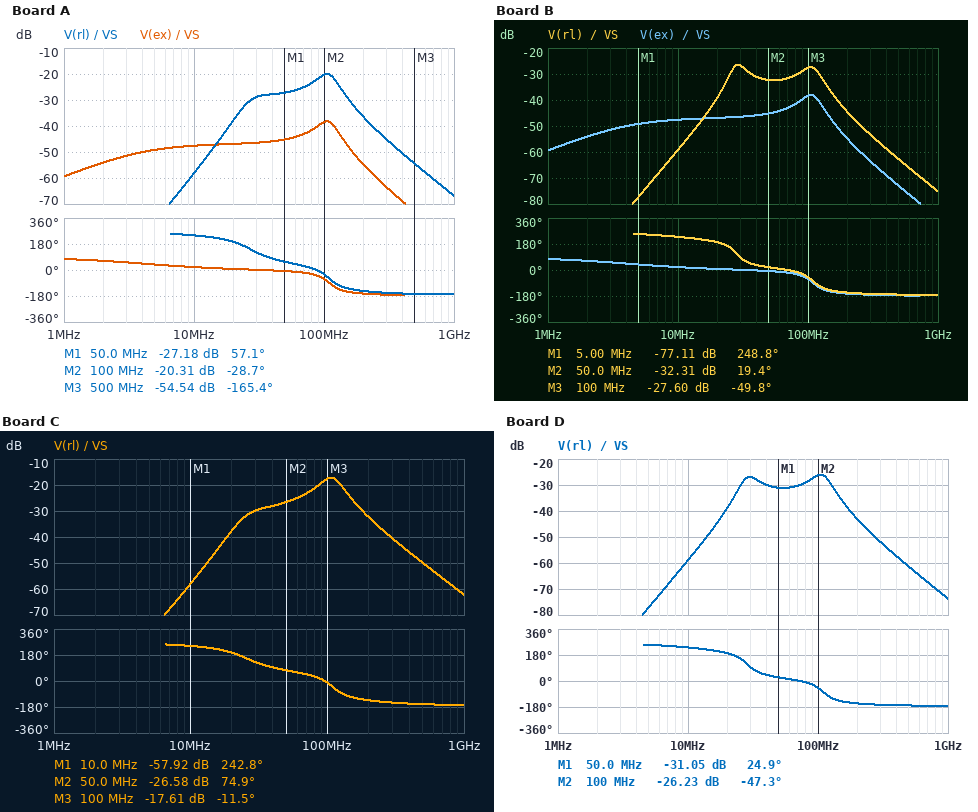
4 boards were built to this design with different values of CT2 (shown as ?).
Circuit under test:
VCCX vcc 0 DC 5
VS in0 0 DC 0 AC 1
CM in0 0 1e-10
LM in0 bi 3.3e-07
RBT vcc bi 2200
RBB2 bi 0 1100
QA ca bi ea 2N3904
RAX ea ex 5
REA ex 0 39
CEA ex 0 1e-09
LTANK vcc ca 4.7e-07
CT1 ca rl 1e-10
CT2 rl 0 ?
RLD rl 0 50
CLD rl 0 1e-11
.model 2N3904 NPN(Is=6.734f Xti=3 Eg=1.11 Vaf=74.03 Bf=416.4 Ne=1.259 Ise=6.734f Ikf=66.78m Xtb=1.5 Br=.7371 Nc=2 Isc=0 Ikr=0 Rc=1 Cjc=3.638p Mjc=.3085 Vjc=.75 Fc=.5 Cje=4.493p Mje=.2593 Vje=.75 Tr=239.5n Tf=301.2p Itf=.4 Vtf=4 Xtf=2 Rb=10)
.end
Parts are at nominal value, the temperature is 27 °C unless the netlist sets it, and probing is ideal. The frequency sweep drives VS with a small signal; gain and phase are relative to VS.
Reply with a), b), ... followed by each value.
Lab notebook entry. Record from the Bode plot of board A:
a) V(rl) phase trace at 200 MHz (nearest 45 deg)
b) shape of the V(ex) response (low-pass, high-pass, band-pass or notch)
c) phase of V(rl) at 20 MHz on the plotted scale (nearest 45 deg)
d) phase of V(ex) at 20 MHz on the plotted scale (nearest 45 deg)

a) -135 deg
b) band-pass
c) 180 deg
d) 0 deg
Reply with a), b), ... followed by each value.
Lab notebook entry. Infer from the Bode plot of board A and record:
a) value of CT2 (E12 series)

a) 39 pF
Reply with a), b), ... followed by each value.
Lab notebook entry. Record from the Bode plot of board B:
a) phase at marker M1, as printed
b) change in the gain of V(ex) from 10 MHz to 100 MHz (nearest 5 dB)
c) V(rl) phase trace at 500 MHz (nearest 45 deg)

a) 248.8 deg
b) 10 dB
c) -180 deg
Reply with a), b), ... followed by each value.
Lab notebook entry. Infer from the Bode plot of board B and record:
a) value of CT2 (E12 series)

a) 120 pF
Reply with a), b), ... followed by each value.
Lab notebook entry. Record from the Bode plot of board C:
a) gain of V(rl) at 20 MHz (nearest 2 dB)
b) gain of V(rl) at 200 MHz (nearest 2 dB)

a) -38 dB
b) -32 dB
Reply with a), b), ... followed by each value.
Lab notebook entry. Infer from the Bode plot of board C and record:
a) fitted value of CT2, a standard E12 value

a) 18 pF
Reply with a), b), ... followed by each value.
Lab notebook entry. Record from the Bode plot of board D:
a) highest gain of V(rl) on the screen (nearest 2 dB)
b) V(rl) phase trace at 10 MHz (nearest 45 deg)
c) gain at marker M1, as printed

a) -26 dB
b) 225 deg
c) -31.05 dB
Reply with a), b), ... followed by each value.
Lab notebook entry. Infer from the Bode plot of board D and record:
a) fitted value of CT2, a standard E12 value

a) 100 pF
